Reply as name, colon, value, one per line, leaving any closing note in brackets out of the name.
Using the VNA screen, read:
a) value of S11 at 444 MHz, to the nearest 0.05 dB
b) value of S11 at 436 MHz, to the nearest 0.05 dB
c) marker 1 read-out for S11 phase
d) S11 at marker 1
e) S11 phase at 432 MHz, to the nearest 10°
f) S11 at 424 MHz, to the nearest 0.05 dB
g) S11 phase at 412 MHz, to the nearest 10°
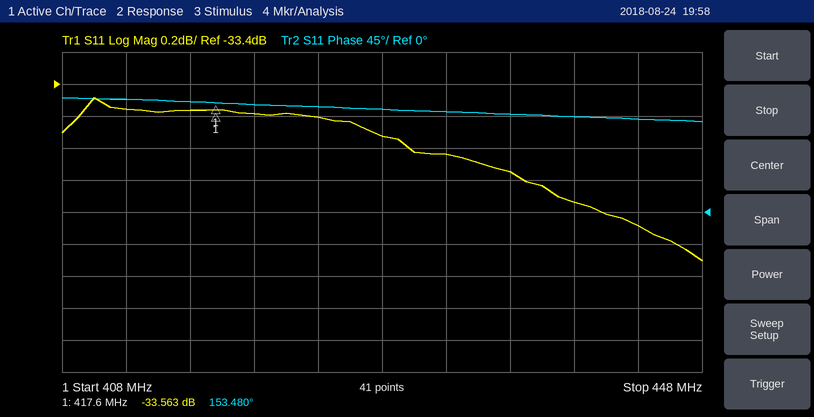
value of S11 at 444 MHz, to the nearest 0.05 dB: -34.30 dB
value of S11 at 436 MHz, to the nearest 0.05 dB: -33.95 dB
marker 1 read-out for S11 phase: 153.480°
S11 at marker 1: -33.563 dB
S11 phase at 432 MHz, to the nearest 10°: 140°
S11 at 424 MHz, to the nearest 0.05 dB: -33.60 dB
S11 phase at 412 MHz, to the nearest 10°: 160°
